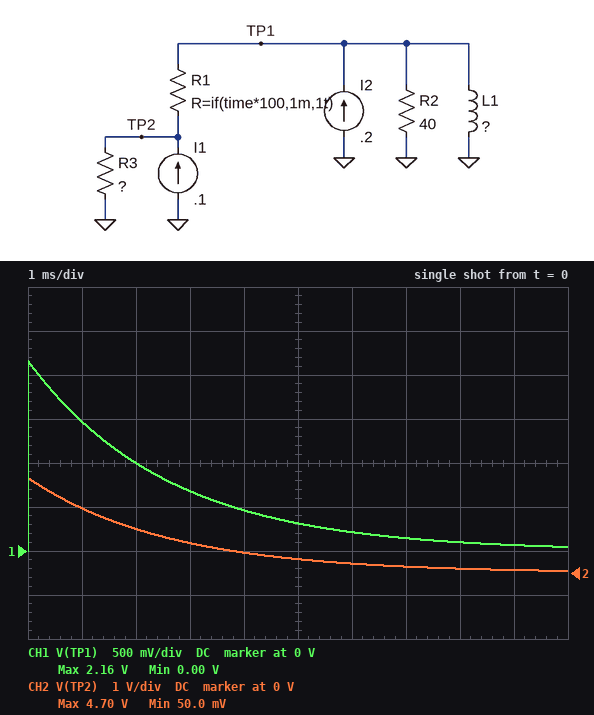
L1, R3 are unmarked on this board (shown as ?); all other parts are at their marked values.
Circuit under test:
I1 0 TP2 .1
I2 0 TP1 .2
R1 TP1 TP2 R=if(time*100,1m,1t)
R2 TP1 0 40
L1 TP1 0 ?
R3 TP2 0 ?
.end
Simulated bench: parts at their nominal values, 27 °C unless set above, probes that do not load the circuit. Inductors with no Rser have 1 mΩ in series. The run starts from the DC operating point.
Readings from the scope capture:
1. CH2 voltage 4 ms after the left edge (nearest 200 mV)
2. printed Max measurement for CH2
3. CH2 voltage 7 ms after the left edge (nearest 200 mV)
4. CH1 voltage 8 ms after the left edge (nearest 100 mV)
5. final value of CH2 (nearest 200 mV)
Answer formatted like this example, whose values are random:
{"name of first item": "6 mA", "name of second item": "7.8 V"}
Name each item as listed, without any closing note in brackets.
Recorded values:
{"CH2 voltage 4 ms after the left edge": "400 mV", "printed Max measurement for CH2": "4.70 V", "CH2 voltage 7 ms after the left edge": "200 mV", "CH1 voltage 8 ms after the left edge": "100 mV", "final value of CH2": "0 V"}
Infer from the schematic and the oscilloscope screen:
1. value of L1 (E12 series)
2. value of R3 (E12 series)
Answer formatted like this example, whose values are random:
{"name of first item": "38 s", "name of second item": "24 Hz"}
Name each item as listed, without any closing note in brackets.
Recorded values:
{"value of L1": "56 mH", "value of R3": "47 Ω"}
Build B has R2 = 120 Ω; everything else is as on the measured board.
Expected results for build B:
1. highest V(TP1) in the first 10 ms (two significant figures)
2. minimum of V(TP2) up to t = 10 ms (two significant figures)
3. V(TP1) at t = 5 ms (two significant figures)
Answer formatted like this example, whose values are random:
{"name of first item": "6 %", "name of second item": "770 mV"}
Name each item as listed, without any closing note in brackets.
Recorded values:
{"highest V(TP1) in the first 10 ms": "3.4 V", "minimum of V(TP2) up to t = 10 ms": "8.5 mV", "V(TP1) at t = 5 ms": "170 mV"}
